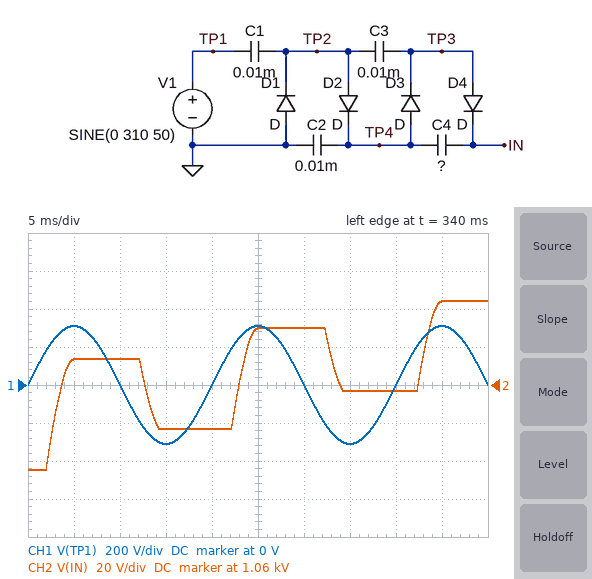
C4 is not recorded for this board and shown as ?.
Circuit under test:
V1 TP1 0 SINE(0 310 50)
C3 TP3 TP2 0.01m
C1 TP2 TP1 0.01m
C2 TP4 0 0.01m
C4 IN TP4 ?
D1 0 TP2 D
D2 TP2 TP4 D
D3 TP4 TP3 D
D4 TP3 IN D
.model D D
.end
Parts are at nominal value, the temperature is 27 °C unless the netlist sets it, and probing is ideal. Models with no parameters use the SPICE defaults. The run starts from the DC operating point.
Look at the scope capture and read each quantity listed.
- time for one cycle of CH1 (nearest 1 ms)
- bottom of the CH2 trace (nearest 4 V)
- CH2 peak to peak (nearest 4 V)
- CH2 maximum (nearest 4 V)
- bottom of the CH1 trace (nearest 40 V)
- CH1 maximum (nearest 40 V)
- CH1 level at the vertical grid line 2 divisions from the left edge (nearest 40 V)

20 ms
1.016 kV
88 V
1.104 kV
-320 V
320 V
0 V
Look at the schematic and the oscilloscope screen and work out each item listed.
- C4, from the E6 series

22 µF
